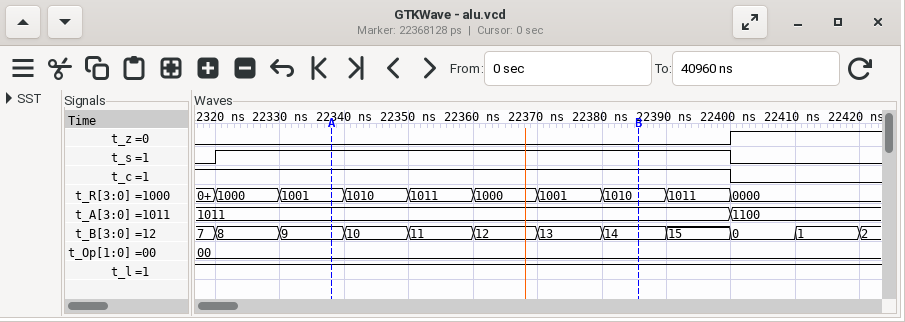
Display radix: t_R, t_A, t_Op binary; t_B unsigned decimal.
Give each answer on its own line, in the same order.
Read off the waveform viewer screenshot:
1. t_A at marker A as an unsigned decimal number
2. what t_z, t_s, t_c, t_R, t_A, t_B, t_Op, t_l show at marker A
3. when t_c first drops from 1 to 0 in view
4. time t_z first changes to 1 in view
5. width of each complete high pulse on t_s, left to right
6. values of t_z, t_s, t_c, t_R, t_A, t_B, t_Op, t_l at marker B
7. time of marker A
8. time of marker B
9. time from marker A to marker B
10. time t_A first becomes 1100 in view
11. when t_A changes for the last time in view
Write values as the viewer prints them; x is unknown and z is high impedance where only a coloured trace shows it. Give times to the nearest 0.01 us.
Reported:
11
t_z=0, t_s=1, t_c=1, t_R=1001, t_A=1011, t_B=9, t_Op=00, t_l=1
22.4 us
22.4 us
0.08 us
t_z=0, t_s=1, t_c=1, t_R=1010, t_A=1011, t_B=14, t_Op=00, t_l=1
22.34 us
22.39 us
0.05 us
22.4 us
22.4 us
